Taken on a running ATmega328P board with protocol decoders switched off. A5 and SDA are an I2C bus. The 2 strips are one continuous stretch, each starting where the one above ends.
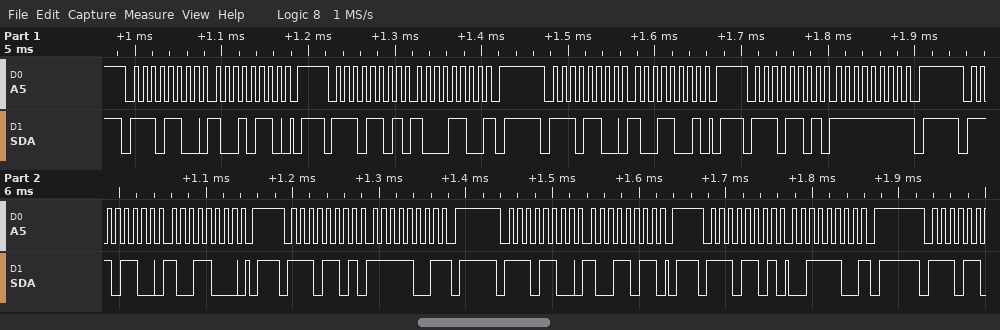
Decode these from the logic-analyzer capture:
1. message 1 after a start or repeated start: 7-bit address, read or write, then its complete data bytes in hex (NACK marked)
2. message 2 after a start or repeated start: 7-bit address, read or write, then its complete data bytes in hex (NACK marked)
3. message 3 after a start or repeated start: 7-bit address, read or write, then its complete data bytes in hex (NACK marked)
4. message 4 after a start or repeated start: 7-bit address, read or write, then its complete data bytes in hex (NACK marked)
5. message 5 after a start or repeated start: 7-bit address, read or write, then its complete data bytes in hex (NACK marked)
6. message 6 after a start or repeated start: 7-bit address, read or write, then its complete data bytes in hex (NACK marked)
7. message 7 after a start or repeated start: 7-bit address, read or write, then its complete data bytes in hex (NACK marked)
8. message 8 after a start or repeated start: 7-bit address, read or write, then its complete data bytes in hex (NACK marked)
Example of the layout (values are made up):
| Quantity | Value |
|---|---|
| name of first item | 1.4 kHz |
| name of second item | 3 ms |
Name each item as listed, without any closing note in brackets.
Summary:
| Quantity | Value |
|---|---|
| message 1 after a start or repeated start: 7-bit address, read or write, then its complete data bytes in hex | 0x76 write: 96 |
| message 2 after a start or repeated start: 7-bit address, read or write, then its complete data bytes in hex | 0x76 read: 8C NACK |
| message 3 after a start or repeated start: 7-bit address, read or write, then its complete data bytes in hex | 0x76 write: 99 |
| message 4 after a start or repeated start: 7-bit address, read or write, then its complete data bytes in hex | 0x76 read: FF NACK |
| message 5 after a start or repeated start: 7-bit address, read or write, then its complete data bytes in hex | 0x76 write: 98 |
| message 6 after a start or repeated start: 7-bit address, read or write, then its complete data bytes in hex | 0x76 read: F9 NACK |
| message 7 after a start or repeated start: 7-bit address, read or write, then its complete data bytes in hex | 0x76 write: 9B |
| message 8 after a start or repeated start: 7-bit address, read or write, then its complete data bytes in hex | 0x76 read: 3C NACK |
